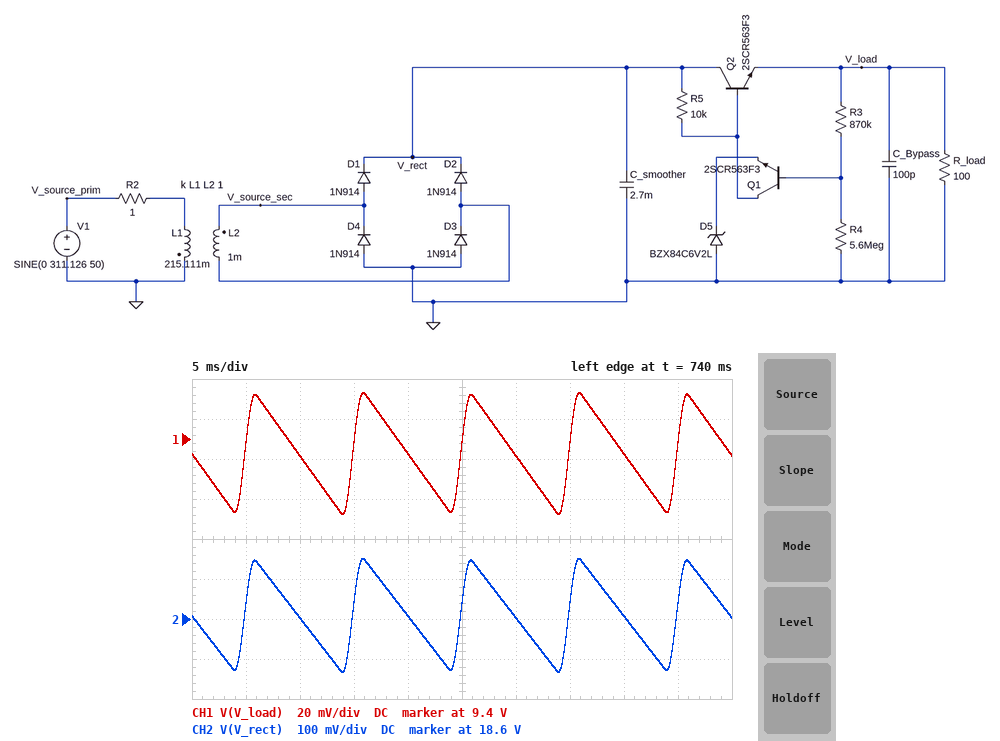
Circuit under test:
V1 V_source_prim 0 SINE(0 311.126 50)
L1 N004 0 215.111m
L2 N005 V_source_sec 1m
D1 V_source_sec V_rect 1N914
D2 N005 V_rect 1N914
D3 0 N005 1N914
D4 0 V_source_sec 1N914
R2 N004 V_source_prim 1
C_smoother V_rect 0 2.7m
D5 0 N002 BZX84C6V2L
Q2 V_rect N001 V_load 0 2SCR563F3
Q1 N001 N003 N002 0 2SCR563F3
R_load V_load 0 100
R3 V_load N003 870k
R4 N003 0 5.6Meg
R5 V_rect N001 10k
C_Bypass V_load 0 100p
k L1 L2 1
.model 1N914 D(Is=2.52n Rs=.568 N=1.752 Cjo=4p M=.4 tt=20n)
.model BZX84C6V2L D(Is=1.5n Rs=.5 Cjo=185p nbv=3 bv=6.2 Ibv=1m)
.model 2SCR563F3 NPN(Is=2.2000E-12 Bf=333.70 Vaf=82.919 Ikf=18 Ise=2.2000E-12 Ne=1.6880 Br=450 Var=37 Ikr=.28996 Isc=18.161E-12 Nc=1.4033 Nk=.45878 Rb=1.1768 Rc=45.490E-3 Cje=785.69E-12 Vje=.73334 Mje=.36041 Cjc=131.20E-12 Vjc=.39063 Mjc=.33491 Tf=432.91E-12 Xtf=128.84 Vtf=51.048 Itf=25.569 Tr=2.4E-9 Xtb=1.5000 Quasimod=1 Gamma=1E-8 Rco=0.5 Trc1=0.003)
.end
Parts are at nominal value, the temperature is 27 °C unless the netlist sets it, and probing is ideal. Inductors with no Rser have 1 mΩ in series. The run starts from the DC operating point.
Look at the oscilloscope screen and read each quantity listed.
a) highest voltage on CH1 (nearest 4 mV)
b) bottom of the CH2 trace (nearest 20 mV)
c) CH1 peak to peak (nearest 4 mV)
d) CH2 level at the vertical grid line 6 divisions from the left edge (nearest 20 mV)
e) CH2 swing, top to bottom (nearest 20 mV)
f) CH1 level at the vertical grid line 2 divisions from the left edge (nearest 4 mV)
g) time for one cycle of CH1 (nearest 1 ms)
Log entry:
9.424 V
18.46 V
60 mV
18.60 V
280 mV
9.392 V
10 ms
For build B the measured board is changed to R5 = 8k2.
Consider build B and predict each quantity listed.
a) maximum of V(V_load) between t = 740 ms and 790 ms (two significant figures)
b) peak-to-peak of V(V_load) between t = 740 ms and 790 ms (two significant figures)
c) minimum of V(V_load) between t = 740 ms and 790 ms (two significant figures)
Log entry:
9.8 V
72 mV
9.7 V
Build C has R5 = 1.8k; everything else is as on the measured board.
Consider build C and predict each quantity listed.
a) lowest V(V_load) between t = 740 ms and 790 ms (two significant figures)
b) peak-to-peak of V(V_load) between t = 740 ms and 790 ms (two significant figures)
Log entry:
13 V
220 mV
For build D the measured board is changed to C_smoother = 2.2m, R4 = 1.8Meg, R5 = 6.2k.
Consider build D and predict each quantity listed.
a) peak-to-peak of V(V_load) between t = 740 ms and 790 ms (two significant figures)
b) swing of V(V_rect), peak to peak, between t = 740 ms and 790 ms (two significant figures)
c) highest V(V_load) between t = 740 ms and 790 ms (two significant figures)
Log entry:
130 mV
430 mV
12 V
